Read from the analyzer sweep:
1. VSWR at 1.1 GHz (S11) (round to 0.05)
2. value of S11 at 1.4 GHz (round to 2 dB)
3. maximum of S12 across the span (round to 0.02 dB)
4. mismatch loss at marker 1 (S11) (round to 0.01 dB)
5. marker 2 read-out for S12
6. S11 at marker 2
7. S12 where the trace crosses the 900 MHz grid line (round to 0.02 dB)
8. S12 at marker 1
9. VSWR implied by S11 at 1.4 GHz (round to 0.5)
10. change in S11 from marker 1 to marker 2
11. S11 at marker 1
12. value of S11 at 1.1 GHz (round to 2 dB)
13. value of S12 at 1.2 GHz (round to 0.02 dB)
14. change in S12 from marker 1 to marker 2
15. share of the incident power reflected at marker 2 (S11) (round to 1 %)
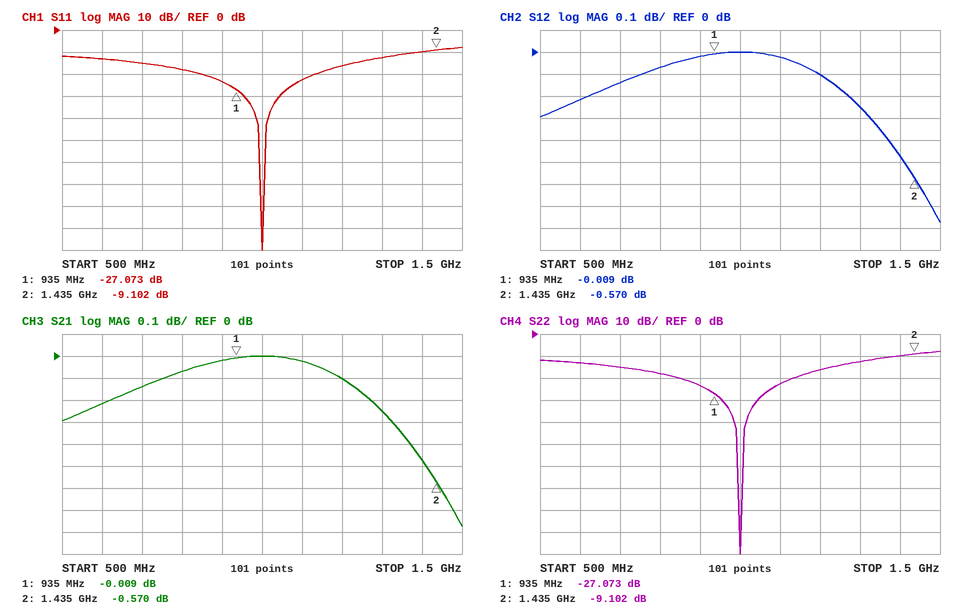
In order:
1.15
-10 dB
0.00 dB
0.01 dB
-0.570 dB
-9.102 dB
-0.02 dB
-0.009 dB
2.0
17.971 dB
-27.073 dB
-22 dB
-0.10 dB
-0.561 dB
12 %
